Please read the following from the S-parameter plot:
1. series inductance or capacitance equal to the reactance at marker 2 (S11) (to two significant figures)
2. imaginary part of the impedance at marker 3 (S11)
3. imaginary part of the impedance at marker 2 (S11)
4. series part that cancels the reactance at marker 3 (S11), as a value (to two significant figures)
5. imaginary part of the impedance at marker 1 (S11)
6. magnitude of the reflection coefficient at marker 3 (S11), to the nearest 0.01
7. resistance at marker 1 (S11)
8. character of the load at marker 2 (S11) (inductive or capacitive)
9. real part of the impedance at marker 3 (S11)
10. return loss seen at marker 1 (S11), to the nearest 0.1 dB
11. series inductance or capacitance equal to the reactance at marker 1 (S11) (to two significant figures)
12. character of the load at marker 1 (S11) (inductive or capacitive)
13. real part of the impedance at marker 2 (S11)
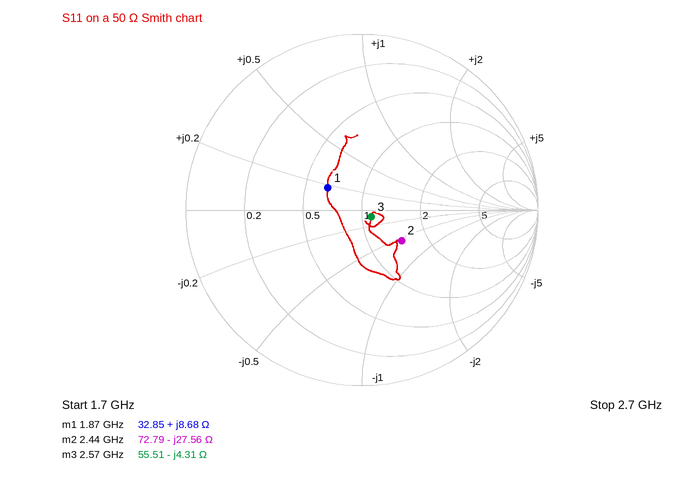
2.4 pF
-4.31 Ω
-27.56 Ω
270 pH
+8.68 Ω
0.07
32.85 Ω
capacitive
55.51 Ω
12.7 dB
740 pH
inductive
72.79 Ω
